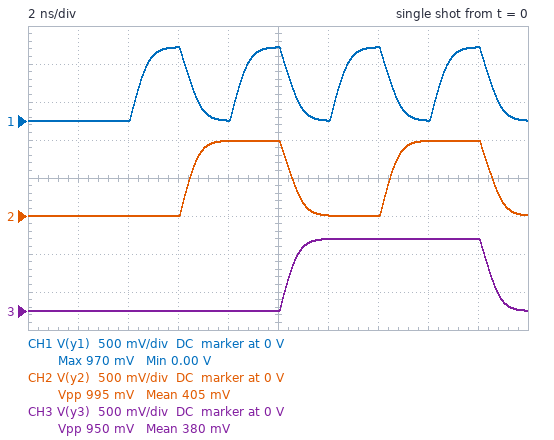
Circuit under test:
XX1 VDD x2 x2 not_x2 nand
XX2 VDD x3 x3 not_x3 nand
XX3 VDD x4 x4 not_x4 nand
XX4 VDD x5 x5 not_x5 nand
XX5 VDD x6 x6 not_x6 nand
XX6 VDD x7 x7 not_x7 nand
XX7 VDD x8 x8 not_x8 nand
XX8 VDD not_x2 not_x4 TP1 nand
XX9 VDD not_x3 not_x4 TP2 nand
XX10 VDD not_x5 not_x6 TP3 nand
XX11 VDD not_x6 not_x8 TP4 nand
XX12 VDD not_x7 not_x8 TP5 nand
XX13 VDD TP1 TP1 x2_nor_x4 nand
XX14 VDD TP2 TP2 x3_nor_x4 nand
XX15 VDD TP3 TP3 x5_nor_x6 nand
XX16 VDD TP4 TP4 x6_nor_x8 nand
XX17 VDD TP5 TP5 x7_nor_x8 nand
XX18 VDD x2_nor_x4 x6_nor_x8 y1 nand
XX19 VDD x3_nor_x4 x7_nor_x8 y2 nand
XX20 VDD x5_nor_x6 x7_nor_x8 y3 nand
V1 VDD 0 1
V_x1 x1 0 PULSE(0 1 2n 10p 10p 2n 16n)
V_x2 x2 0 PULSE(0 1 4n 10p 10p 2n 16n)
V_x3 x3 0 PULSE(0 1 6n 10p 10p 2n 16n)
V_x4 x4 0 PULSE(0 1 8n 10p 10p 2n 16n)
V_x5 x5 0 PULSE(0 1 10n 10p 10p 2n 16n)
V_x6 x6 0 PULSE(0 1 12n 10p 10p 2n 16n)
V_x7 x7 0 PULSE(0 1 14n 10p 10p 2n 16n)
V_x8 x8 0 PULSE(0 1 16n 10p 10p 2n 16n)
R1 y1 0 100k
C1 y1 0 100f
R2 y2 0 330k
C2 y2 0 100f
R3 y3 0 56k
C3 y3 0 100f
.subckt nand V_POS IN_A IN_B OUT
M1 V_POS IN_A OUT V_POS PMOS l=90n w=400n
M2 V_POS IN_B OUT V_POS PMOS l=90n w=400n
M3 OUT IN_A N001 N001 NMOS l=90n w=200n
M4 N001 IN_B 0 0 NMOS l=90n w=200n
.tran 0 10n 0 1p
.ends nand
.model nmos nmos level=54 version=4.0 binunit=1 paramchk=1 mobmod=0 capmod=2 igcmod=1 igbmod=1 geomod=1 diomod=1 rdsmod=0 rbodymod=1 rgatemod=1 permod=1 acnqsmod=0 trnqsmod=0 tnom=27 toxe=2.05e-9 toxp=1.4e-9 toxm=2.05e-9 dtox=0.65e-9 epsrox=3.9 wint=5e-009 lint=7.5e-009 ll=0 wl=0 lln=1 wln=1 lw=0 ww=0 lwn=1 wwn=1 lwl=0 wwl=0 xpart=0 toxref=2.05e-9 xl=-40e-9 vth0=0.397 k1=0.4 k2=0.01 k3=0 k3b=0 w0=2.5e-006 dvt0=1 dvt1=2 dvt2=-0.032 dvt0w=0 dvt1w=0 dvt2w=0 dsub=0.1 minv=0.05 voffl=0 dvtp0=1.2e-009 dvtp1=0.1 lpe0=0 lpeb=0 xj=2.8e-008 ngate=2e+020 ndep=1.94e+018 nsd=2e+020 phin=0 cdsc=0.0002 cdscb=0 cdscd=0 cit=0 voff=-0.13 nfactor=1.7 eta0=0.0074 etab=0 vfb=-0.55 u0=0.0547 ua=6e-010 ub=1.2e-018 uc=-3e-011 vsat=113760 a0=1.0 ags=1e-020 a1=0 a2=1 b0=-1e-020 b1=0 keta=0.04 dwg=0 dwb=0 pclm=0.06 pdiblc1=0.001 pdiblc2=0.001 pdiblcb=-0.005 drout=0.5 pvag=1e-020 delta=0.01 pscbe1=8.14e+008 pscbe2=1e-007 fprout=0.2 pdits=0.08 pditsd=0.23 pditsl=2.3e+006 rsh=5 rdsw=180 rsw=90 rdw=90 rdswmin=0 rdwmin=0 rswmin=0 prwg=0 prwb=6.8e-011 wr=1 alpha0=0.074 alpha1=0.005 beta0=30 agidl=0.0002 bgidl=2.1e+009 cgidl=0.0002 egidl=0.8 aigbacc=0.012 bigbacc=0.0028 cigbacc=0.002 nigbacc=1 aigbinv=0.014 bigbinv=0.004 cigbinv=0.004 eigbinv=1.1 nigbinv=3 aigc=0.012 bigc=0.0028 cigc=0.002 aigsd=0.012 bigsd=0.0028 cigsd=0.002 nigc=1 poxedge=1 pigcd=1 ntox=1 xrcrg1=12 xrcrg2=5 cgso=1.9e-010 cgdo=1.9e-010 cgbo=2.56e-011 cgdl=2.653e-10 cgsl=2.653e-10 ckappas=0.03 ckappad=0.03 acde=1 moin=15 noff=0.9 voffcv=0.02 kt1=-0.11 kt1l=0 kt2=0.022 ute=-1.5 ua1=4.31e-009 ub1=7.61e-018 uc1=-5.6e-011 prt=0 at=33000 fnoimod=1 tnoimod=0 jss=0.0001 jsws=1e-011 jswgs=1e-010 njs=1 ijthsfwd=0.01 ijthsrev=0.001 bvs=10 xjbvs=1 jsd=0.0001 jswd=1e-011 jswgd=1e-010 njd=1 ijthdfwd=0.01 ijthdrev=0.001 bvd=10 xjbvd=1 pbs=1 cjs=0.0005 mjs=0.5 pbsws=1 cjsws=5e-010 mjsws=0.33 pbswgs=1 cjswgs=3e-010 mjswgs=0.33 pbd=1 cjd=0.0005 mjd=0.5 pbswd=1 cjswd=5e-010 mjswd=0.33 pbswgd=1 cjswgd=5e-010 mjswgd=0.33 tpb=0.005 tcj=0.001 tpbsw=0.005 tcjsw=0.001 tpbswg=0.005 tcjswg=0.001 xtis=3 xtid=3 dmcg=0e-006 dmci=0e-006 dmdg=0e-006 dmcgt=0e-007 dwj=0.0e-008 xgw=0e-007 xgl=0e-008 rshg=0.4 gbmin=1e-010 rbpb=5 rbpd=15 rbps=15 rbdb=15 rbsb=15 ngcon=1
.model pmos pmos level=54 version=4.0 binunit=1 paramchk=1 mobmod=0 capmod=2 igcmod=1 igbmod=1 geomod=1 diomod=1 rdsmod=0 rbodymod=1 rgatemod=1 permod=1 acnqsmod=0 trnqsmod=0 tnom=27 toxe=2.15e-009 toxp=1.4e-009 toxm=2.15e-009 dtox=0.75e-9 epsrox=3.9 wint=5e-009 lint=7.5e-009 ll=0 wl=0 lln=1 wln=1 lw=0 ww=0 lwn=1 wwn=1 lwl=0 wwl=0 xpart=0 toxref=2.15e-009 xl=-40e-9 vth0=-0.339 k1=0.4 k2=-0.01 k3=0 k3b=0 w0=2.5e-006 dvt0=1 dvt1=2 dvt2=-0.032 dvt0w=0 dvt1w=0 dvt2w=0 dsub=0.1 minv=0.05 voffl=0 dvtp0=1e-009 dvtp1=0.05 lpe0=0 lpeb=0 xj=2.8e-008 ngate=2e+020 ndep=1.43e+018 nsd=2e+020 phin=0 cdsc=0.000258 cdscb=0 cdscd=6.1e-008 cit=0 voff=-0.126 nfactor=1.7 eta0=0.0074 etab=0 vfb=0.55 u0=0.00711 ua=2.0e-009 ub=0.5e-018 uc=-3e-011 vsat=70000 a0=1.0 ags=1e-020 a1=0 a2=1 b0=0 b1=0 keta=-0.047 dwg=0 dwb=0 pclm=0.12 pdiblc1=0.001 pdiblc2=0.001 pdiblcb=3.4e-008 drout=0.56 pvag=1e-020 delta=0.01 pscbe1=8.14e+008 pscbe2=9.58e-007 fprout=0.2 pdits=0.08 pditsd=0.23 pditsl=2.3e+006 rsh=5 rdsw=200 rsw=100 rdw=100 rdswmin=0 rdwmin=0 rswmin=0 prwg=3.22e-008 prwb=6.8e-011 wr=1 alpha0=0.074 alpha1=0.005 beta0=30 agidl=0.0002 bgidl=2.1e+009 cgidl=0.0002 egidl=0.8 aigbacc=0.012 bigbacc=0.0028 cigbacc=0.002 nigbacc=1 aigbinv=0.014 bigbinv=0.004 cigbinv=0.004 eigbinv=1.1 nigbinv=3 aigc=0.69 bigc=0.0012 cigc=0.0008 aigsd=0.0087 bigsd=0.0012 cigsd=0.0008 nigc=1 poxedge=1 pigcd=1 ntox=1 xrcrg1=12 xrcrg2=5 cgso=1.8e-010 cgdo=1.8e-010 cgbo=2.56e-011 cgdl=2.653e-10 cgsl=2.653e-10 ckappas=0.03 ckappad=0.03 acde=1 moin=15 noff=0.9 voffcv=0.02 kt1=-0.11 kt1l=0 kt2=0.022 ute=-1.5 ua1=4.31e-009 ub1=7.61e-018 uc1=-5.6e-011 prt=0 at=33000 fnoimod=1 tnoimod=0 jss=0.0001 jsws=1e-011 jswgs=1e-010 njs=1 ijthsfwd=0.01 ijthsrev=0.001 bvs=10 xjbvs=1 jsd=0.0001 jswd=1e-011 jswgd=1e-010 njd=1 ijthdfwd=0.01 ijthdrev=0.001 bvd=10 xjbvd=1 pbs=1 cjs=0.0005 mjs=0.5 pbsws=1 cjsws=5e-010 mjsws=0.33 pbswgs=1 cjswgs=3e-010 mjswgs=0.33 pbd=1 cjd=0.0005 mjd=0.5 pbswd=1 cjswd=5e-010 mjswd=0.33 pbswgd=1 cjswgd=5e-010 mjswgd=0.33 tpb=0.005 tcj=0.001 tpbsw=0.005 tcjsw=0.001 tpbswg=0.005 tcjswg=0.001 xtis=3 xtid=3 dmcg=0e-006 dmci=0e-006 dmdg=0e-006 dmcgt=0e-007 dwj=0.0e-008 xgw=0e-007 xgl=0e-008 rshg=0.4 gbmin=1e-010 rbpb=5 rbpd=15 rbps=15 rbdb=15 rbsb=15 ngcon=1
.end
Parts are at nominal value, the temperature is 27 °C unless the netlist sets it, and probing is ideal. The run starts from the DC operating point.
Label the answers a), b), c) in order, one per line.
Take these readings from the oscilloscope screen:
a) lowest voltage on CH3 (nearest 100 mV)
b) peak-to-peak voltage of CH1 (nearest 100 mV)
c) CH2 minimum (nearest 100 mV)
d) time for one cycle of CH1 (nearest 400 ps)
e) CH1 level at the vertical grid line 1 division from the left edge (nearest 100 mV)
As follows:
a) 0 V
b) 1.0 V
c) 0 V
d) 4.0 ns
e) 0 V
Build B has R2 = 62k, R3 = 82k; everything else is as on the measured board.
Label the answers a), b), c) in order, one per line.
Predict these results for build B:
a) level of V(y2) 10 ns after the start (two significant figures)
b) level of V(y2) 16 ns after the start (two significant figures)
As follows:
a) 960 mV
b) 950 mV
